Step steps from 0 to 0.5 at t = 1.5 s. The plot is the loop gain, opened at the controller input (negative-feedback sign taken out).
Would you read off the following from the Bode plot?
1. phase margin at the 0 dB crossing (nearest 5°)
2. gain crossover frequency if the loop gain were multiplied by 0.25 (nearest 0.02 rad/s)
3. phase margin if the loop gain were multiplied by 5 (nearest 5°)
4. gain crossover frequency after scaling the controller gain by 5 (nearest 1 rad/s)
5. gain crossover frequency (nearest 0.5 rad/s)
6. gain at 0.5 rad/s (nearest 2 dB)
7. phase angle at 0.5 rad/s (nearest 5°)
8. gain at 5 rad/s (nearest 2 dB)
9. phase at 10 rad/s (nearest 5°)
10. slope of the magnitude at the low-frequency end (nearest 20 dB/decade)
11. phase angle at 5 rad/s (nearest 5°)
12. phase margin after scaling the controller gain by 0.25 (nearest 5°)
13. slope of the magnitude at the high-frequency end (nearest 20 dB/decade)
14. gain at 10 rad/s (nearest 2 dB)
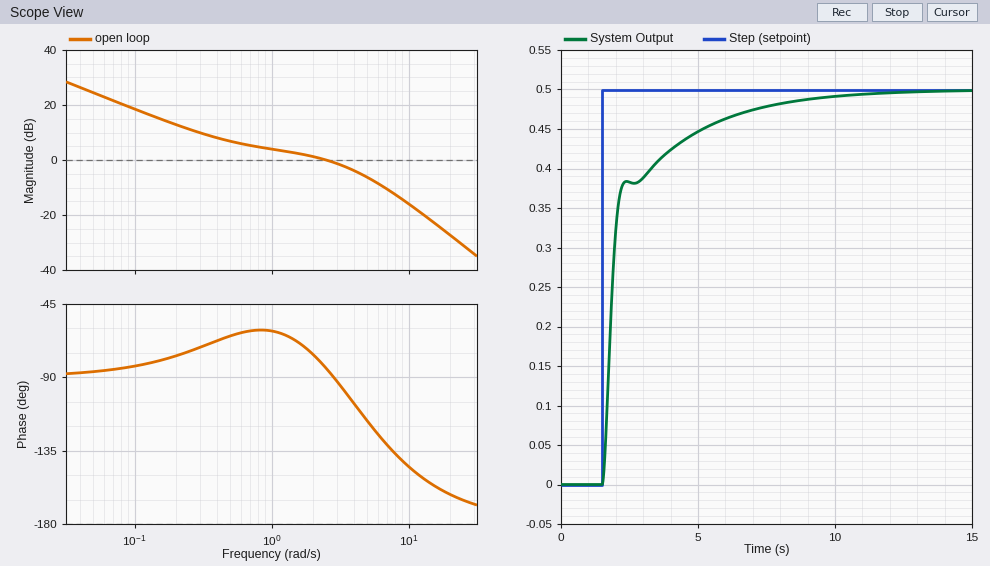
95°
0.22 rad/s
40°
9 rad/s
2.5 rad/s
6 dB
-65°
-6 dB
-145°
-20 dB/decade
-115°
105°
-40 dB/decade
-16 dB
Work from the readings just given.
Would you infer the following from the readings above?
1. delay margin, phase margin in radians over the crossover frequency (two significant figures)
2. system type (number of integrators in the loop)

0.66 s
1
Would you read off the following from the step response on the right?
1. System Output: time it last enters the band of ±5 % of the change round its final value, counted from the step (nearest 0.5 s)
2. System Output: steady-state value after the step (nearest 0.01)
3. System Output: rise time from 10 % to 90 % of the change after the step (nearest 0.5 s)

5.5 s
0.50
3.5 s
